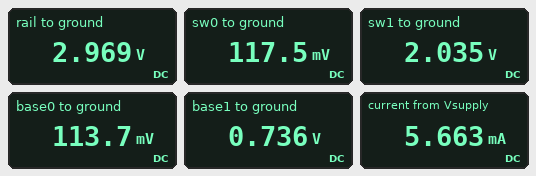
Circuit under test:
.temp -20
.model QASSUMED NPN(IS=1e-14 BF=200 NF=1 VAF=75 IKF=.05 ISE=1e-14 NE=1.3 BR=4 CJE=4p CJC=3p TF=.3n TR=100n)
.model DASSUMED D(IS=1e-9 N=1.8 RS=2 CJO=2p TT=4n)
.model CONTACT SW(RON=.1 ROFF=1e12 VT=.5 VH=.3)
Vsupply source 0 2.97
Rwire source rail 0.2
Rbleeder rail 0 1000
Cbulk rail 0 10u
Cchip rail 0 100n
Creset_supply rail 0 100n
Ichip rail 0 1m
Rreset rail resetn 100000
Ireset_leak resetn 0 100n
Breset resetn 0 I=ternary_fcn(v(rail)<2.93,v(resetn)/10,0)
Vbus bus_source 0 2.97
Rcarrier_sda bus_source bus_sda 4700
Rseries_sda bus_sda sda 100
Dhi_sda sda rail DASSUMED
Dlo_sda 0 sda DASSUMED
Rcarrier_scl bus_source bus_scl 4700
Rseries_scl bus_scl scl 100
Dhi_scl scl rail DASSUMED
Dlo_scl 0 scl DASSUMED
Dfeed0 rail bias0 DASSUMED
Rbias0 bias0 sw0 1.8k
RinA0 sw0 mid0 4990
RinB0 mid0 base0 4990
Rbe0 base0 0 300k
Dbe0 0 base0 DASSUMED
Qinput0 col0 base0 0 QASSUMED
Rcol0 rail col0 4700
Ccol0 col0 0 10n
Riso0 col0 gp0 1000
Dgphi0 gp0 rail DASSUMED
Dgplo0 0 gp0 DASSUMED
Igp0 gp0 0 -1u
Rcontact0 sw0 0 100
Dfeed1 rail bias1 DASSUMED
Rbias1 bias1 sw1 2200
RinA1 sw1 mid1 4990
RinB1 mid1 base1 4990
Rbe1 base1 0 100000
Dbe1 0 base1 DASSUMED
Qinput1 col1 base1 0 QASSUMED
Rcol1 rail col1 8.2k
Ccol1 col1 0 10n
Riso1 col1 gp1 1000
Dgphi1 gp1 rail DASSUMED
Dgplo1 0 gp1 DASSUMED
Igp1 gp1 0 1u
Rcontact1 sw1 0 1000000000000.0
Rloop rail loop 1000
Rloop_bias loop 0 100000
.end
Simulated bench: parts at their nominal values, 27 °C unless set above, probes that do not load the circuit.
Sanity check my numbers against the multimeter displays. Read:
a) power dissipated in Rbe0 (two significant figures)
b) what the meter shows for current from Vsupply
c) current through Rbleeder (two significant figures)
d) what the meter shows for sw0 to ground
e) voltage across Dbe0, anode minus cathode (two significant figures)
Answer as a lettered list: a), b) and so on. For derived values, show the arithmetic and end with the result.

a) (113.7 mV)^2 / 300 kΩ = 43 nW
b) 5.663 mA
c) (2.969 V) / 1 kΩ = 3.0 mA
d) 117.5 mV
e) 0 V - 113.7 mV = -110 mV
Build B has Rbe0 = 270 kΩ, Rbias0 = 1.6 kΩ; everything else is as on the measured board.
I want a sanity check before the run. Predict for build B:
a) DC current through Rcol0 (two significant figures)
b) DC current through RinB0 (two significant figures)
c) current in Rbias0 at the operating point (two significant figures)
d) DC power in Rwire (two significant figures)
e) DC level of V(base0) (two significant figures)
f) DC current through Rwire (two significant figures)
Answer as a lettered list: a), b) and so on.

a) 1.0 µA
b) 470 nA
c) 1.3 mA
d) 6.7 µW
e) 130 mV
f) 5.8 mA
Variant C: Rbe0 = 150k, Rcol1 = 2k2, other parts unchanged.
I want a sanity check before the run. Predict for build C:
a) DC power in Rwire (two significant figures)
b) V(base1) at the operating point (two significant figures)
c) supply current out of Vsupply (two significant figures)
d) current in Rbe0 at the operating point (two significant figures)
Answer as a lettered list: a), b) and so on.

a) 8.8 µW
b) 750 mV
c) 6.6 mA
d) 730 nA
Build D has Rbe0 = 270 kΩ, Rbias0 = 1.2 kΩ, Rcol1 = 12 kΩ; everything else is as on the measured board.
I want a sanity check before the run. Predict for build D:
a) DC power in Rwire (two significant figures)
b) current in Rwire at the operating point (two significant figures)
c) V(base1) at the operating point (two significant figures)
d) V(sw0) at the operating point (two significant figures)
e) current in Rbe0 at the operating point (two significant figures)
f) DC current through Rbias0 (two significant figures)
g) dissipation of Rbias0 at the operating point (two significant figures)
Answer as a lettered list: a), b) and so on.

a) 7.4 µW
b) 6.1 mA
c) 730 mV
d) 170 mV
e) 610 nA
f) 1.7 mA
g) 3.5 mW
